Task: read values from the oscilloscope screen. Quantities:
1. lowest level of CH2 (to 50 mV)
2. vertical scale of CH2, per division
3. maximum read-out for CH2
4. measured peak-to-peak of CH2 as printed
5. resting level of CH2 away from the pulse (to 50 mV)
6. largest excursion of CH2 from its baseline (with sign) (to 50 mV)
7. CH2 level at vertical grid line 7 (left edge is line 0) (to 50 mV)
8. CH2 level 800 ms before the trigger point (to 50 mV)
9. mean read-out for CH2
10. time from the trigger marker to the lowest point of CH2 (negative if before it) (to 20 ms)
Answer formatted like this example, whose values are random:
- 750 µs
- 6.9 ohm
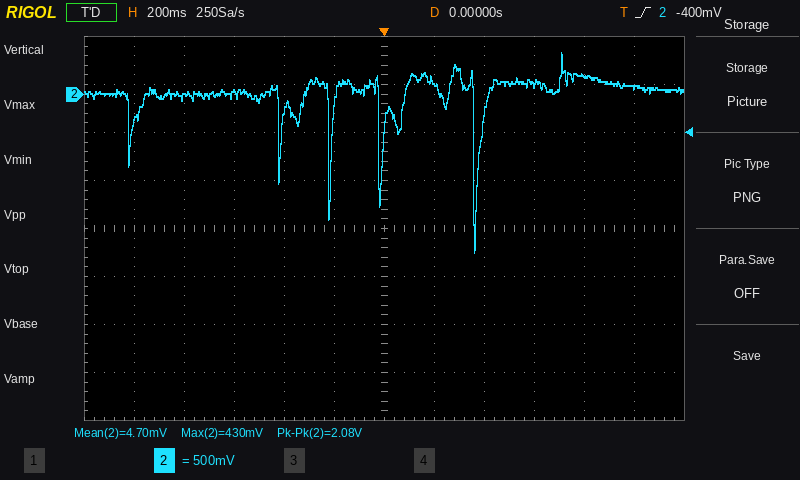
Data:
- -1.65 V
- 500 mV
- 430 mV
- 2.08 V
- 50 mV
- -1.70 V
- 150 mV
- -50 mV
- 4.70 mV
- +360 ms
